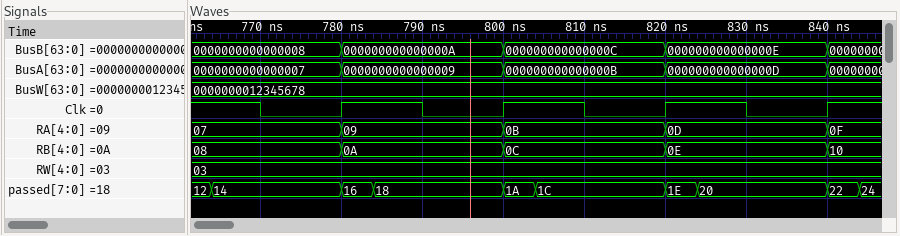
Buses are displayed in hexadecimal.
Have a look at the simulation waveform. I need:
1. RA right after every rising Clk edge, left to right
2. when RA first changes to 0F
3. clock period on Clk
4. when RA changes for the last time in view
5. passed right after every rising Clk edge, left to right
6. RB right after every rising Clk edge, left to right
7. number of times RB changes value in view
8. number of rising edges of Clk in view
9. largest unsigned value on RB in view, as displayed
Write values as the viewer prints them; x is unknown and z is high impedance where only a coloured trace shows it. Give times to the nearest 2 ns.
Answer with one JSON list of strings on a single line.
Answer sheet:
["09, 0B, 0D, 0F", "840 ns", "20 ns", "840 ns", "16, 1A, 1E, 22", "0A, 0C, 0E, 10", "4", "4", "10"]
